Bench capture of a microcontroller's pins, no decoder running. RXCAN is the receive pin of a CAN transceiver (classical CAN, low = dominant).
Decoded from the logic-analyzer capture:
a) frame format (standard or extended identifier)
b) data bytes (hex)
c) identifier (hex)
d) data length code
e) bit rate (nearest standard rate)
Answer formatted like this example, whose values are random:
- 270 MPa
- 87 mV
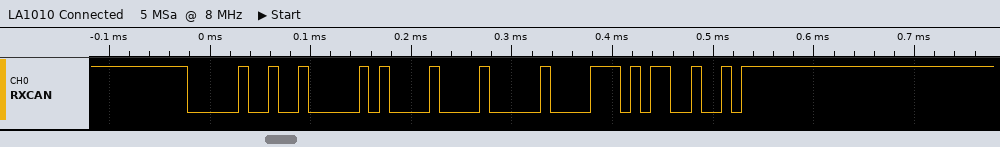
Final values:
- standard
- 10 80
- 0x012
- 2
- 100 kbit/s
